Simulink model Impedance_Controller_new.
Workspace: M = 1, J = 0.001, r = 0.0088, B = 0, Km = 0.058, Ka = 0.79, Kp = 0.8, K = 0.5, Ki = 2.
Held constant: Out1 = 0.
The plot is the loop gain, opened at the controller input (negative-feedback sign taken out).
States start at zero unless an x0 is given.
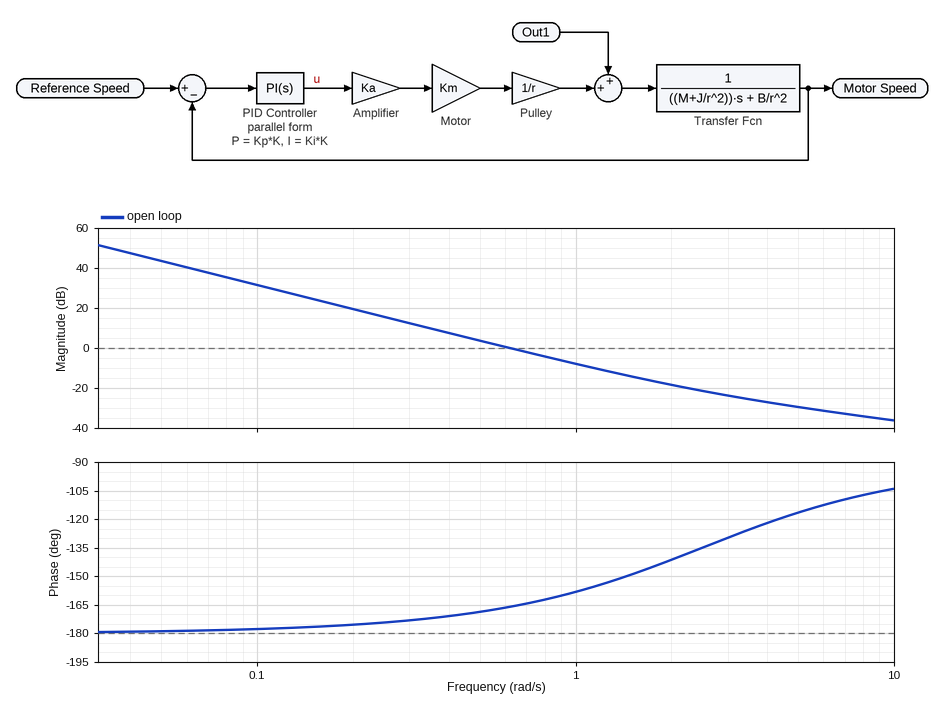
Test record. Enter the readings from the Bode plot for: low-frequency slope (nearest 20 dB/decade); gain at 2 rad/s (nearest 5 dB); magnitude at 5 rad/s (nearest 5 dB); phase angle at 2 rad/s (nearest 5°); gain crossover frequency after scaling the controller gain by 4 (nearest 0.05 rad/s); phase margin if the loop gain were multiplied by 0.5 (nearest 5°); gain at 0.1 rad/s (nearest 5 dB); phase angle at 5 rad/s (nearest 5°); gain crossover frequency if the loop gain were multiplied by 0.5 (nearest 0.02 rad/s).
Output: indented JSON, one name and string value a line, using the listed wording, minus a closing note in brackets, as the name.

{
  "low-frequency slope": "-40 dB/decade",
  "gain at 2 rad/s": "-20 dB",
  "magnitude at 5 rad/s": "-30 dB",
  "phase angle at 2 rad/s": "-140°",
  "gain crossover frequency after scaling the controller gain by 4": "1.30 rad/s",
  "phase margin if the loop gain were multiplied by 0.5": "10°",
  "gain at 0.1 rad/s": "30 dB",
  "phase angle at 5 rad/s": "-115°",
  "gain crossover frequency if the loop gain were multiplied by 0.5": "0.44 rad/s"
}
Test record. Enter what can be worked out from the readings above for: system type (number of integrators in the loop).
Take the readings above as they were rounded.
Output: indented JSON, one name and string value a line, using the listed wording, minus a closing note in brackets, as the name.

{
  "system type": "2"
}
